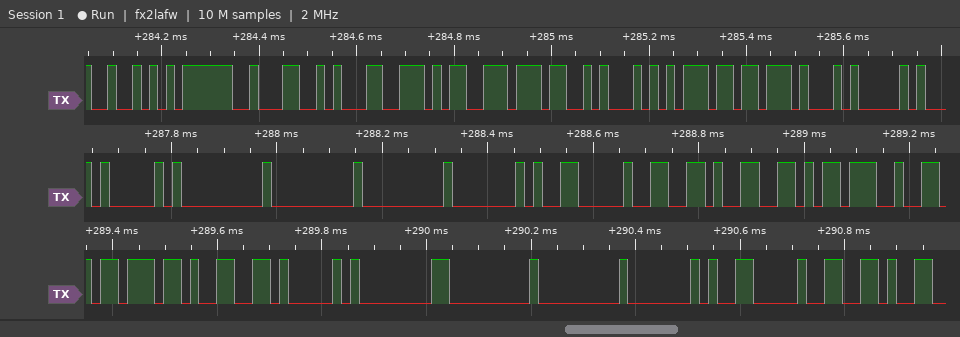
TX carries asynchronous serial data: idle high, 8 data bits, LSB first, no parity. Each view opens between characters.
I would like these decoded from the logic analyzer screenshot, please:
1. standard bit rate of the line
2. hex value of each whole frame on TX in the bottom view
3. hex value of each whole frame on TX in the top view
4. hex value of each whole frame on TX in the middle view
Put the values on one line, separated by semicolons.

57600 baud; BB, 99, 41, 80, 00, 00, 40, 06, 66; 52, 3F, 4C, CC, CD, 37, 51, B7, 17, 41; 41, 00, 00, 00, 40, 06, 66, 66, 3B
